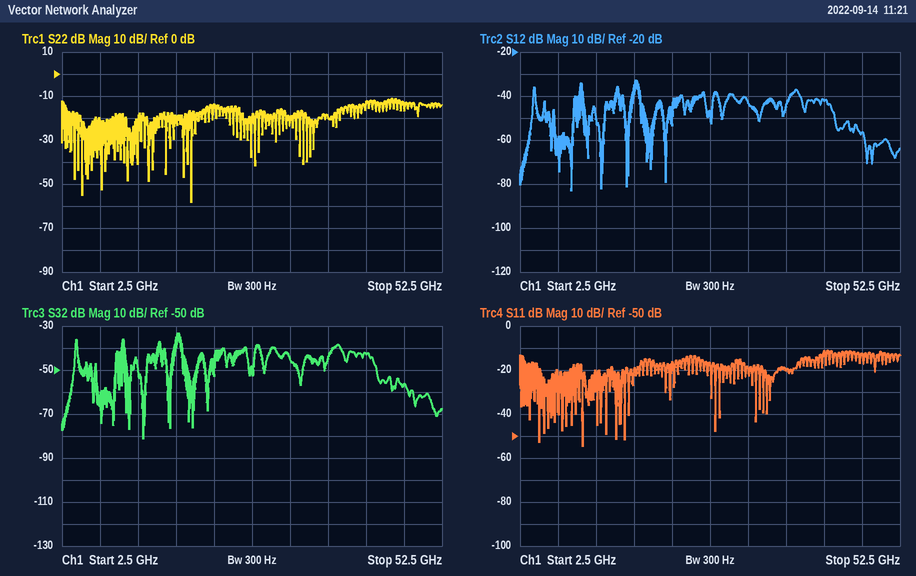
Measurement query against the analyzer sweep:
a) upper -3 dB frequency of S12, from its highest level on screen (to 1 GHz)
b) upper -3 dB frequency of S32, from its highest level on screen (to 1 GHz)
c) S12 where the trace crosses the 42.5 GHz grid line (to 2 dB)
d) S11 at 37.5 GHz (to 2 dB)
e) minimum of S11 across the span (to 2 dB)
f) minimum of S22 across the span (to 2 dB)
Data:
18 GHz
18 GHz
-42 dB
-20 dB
-54 dB
-58 dB
